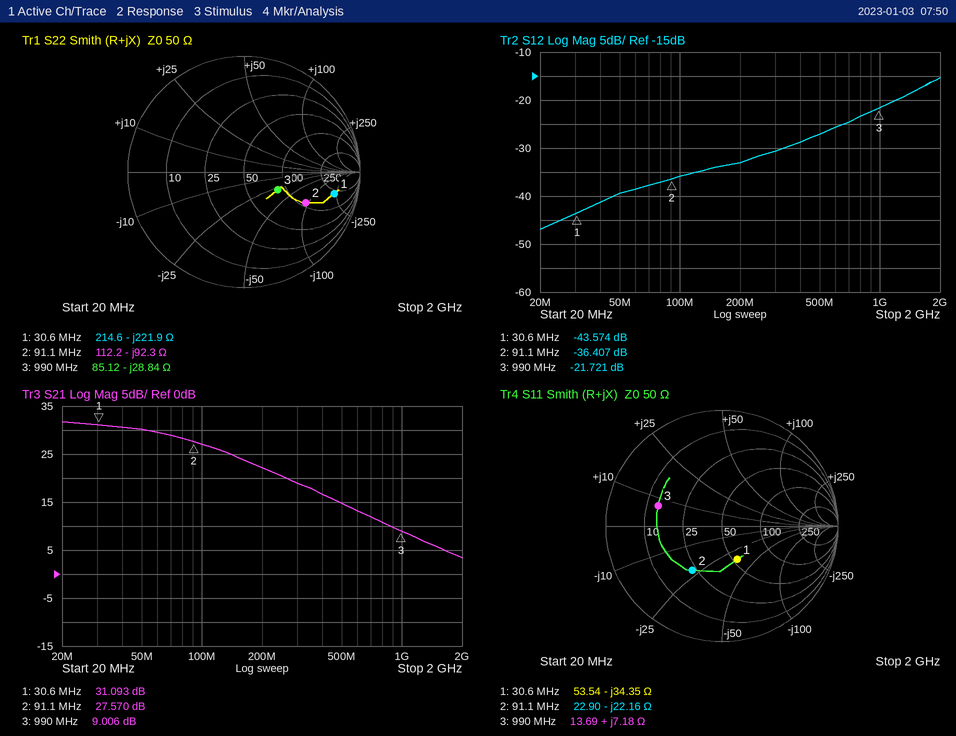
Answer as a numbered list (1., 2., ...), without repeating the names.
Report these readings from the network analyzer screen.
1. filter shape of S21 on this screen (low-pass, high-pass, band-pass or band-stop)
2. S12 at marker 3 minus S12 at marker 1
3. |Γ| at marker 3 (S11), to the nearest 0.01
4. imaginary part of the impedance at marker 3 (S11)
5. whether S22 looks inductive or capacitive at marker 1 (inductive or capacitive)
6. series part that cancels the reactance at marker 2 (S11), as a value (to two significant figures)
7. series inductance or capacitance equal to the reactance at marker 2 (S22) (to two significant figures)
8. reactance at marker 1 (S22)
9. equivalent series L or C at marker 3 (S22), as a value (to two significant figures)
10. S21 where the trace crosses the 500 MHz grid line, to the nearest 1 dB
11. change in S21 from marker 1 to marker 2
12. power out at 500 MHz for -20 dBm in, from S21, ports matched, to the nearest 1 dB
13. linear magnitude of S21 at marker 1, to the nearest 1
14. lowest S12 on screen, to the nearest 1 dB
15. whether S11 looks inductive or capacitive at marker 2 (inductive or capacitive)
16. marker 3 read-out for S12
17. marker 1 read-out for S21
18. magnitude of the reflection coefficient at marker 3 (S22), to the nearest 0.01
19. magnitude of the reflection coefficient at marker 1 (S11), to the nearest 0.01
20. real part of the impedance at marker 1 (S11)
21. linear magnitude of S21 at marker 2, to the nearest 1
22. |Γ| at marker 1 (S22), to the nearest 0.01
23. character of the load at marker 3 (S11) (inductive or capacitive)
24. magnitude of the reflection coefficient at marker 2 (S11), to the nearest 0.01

1. low-pass
2. 21.853 dB
3. 0.58
4. +7.18 Ω
5. capacitive
6. 39 nH
7. 19 pF
8. -221.9 Ω
9. 5.6 pF
10. 15 dB
11. -3.523 dB
12. -5 dBm
13. 36
14. -47 dB
15. capacitive
16. -21.721 dB
17. 31.093 dB
18. 0.33
19. 0.32
20. 53.54 Ω
21. 24
22. 0.80
23. inductive
24. 0.46
